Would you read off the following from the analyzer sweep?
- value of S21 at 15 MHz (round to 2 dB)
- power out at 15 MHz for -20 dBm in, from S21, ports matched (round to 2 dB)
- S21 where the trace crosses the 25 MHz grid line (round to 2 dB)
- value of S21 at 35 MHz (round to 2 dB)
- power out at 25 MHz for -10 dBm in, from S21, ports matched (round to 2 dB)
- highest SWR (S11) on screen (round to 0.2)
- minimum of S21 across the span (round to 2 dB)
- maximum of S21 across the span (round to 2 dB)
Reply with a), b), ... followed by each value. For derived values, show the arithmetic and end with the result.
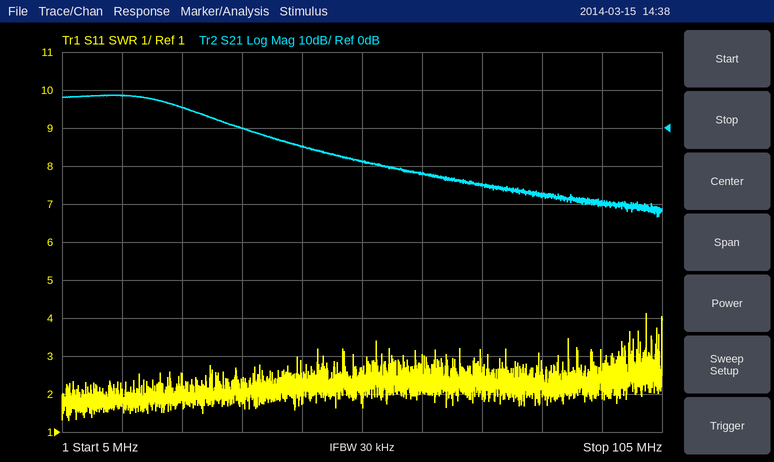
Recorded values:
a) 8 dB
b) -20 dBm + (8 dB) = -12 dBm
c) 6 dB
d) 0 dB
e) -10 dBm + (6 dB) = -4 dBm
f) 4.2
g) -24 dB
h) 8 dB
